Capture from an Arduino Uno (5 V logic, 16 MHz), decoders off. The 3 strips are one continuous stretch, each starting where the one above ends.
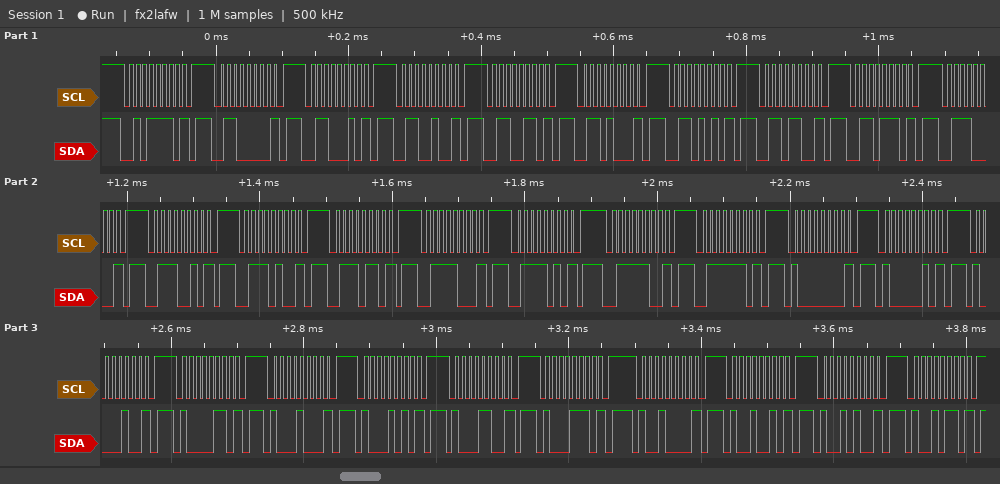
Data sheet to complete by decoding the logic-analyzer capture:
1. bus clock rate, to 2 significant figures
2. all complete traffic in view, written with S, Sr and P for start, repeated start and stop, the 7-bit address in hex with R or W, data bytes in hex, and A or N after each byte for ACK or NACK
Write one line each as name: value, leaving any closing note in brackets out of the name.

bus clock rate, to 2 significant figures: 100 kHz
all complete traffic in view, written with S, Sr and P for start, repeated start and stop, the 7-bit address in hex with R or W, data bytes in hex, and A or N after each byte for ACK or NACK: S 2FW N P S 30W N P S 31W N P S 32W N P S 33W N P S 34W N P S 35W N P S 36W N P S 37W N P S 38W N P S 39W N P S 3AW N P S 3BW N P S 3CW N P S 3DW N P S 3EW N P S 3FW N P S 40W N P S 41W N P S 42W N P S 43W N P S 44W N P S 45W N P S 46W N P S 47W N P S 48W N P S 49W N P S 4AW N P S 4BW N P
